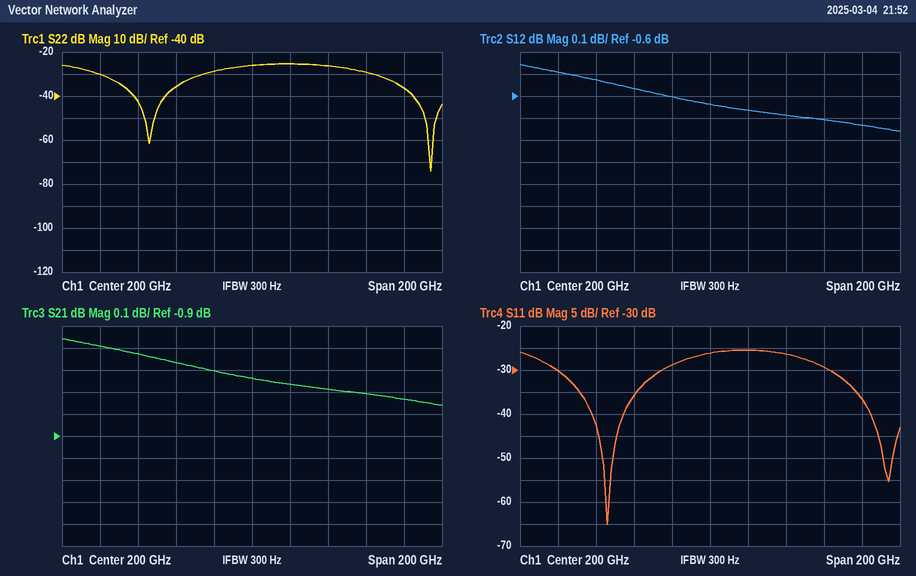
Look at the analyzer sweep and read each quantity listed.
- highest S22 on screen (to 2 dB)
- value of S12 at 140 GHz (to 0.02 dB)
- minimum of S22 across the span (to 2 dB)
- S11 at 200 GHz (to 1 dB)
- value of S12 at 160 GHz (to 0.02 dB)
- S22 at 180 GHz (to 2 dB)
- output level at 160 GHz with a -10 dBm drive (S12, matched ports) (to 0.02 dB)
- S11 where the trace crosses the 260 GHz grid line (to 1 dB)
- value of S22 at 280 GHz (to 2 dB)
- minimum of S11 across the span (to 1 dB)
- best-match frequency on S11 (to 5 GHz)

-26 dB
-0.52 dB
-74 dB
-26 dB
-0.56 dB
-28 dB
-10.56 dBm
-29 dB
-36 dB
-65 dB
145 GHz
